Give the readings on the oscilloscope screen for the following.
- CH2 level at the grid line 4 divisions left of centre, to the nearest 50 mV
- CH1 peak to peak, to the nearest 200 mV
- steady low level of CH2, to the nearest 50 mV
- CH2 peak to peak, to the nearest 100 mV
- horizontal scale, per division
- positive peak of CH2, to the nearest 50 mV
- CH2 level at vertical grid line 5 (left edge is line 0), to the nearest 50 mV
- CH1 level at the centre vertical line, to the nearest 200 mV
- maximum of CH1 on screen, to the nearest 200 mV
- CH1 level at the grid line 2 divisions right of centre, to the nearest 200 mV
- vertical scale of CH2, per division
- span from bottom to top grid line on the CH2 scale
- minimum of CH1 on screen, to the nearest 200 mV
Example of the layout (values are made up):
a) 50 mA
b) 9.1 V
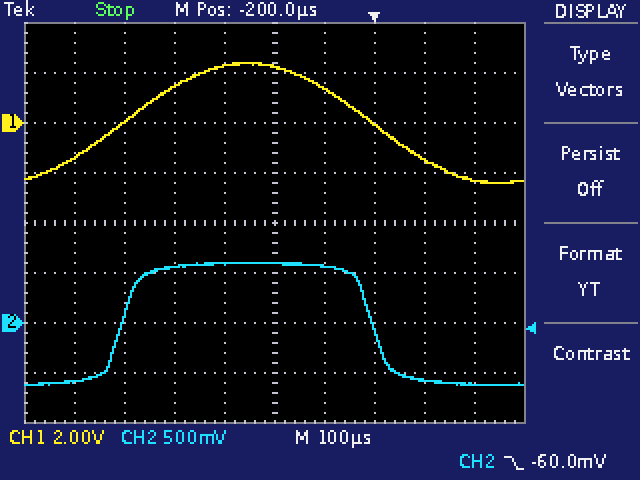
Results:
a) -600 mV
b) 4.8 V
c) -600 mV
d) 1.20 V
e) 100 µs
f) 600 mV
g) 600 mV
h) 2.2 V
i) 2.4 V
j) 0.0 V
k) 500 mV
l) 4 V
m) -2.4 V
